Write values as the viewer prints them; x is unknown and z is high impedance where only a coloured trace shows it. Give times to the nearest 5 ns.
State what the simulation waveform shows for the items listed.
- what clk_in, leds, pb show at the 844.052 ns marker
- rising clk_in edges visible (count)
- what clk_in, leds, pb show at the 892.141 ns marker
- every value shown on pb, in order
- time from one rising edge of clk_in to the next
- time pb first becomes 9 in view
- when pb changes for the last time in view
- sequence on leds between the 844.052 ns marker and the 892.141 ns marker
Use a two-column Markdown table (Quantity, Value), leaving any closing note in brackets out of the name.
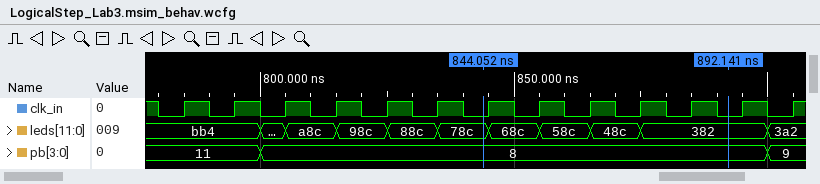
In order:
| Quantity | Value |
|---|---|
| what clk_in, leds, pb show at the 844.052 ns marker | clk_in=0, leds=78c, pb=8 |
| rising clk_in edges visible | 13 |
| what clk_in, leds, pb show at the 892.141 ns marker | clk_in=0, leds=382, pb=8 |
| every value shown on pb, in order | 11, 8, 9 |
| time from one rising edge of clk_in to the next | 10 ns |
| time pb first becomes 9 in view | 900 ns |
| when pb changes for the last time in view | 900 ns |
| sequence on leds between the 844.052 ns marker and the 892.141 ns marker | 78c, 68c, 58c, 48c, 382 |
